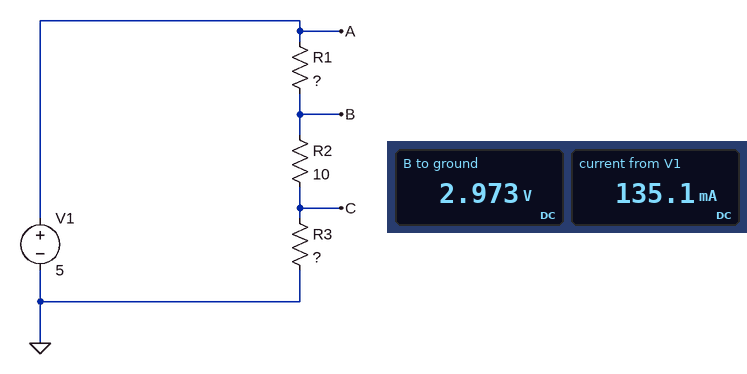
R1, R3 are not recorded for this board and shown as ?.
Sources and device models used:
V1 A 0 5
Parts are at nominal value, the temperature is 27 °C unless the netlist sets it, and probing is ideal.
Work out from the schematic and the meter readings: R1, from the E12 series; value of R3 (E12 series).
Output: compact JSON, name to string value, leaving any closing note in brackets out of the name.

{"R1, from the E12 series": "15 Ω", "value of R3": "12 Ω"}
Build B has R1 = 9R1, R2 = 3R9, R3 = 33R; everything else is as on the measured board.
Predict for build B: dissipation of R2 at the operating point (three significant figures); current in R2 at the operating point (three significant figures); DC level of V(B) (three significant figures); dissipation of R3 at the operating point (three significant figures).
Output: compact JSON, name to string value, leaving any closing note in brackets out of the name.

{"dissipation of R2 at the operating point": "46.1 mW", "current in R2 at the operating point": "109 mA", "DC level of V(B)": "4.01 V", "dissipation of R3 at the operating point": "390 mW"}
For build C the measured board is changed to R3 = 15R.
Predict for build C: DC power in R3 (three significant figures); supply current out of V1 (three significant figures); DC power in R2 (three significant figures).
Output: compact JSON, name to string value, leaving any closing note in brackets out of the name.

{"DC power in R3": "234 mW", "supply current out of V1": "125 mA", "DC power in R2": "156 mW"}
